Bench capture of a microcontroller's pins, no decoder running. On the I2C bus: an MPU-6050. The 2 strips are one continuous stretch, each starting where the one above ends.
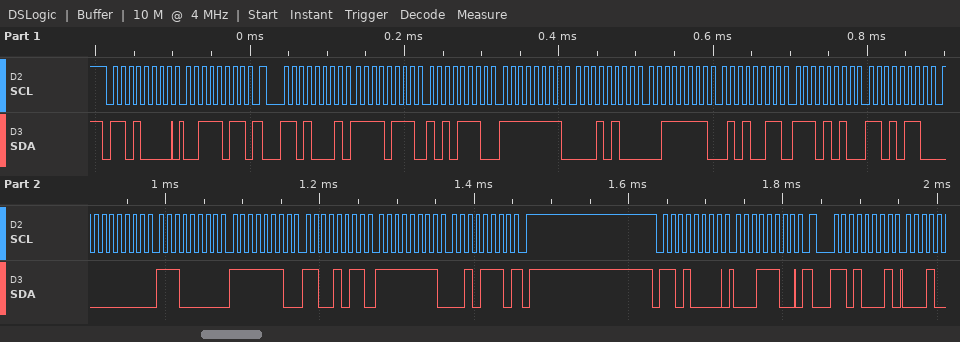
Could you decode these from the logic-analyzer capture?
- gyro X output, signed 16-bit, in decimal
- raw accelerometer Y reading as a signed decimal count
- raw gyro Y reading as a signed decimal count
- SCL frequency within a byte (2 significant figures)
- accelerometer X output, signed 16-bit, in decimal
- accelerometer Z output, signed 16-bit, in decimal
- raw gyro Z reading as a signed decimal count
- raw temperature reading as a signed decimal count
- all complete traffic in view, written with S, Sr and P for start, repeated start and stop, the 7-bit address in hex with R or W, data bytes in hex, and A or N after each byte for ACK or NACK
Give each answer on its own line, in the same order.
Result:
224
-236
-309
100 kHz
-2130
16211
-210
-5418
S 68W A 3B A Sr 68R A F7 A AE A FF A 14 A 3F A 53 A EA A D6 A 00 A E0 A FE A CB A FF A 2E N P S 68W A 1C A Sr 68R A
